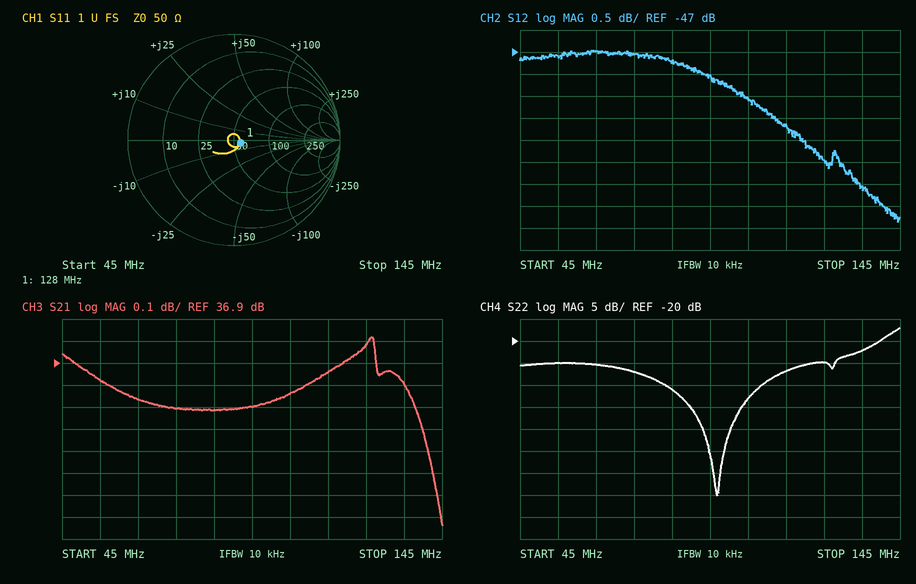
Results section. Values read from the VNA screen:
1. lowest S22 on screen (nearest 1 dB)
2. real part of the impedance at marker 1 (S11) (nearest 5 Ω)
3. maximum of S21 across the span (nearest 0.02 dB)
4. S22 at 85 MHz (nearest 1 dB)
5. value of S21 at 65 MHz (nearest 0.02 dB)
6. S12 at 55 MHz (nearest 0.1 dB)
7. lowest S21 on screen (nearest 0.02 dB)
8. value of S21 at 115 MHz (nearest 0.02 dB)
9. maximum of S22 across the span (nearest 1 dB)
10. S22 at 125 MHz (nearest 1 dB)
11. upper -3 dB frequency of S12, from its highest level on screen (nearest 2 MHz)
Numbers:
-55 dB
55 Ω
37.02 dB
-31 dB
36.74 dB
-47.1 dB
36.16 dB
36.86 dB
-17 dB
-25 dB
134 MHz
